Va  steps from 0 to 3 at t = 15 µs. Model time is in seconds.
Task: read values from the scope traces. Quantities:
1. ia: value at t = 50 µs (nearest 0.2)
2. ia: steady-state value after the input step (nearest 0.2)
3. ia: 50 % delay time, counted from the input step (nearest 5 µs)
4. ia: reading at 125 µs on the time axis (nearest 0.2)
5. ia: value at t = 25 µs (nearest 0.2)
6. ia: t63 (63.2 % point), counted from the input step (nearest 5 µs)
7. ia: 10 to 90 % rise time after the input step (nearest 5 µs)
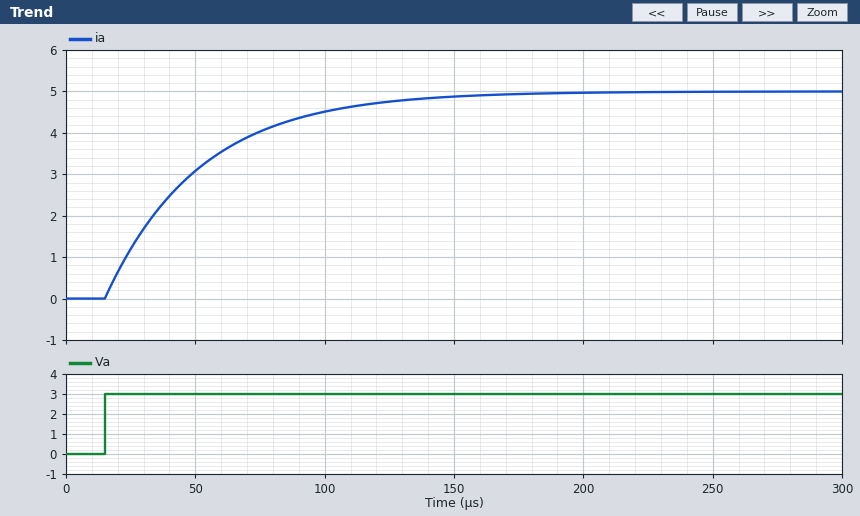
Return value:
3.0
5.0
25 µs
4.8
1.2
35 µs
80 µs
